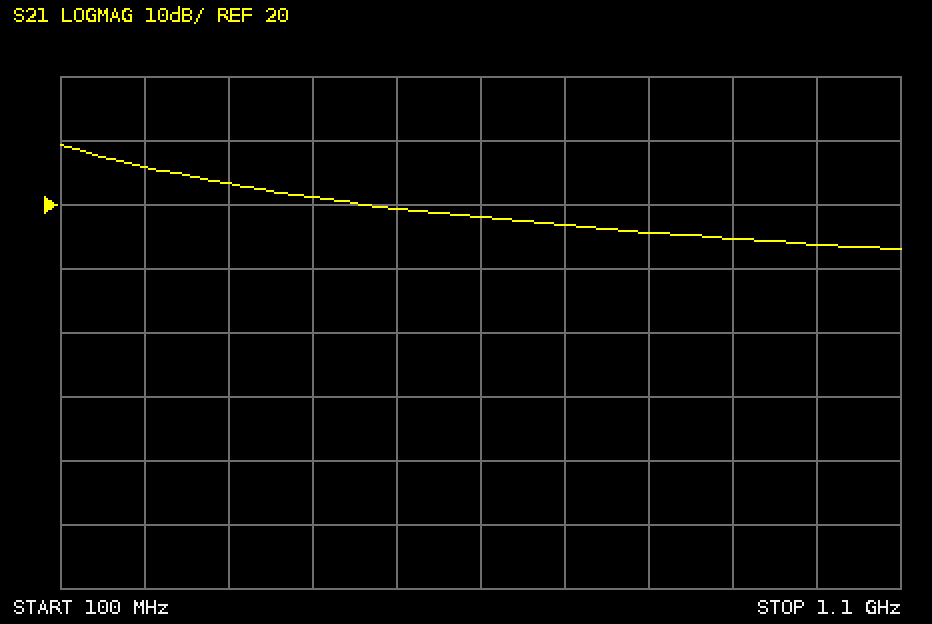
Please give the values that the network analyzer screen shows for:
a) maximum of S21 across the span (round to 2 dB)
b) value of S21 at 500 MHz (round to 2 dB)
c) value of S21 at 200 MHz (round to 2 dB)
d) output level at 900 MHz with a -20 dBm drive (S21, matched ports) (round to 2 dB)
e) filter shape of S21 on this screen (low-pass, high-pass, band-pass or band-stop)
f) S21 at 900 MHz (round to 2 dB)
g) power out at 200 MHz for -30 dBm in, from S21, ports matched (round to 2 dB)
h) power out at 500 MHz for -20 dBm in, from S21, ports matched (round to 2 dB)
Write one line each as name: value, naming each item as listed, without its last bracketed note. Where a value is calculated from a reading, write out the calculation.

maximum of S21 across the span: 30 dB
value of S21 at 500 MHz: 20 dB
value of S21 at 200 MHz: 26 dB
output level at 900 MHz with a -20 dBm drive (S21, matched ports): -20 dBm + (14 dB) = -6 dBm
filter shape of S21 on this screen: low-pass
S21 at 900 MHz: 14 dB
power out at 200 MHz for -30 dBm in, from S21, ports matched: -30 dBm + (26 dB) = -4 dBm
power out at 500 MHz for -20 dBm in, from S21, ports matched: -20 dBm + (20 dB) = 0 dBm
